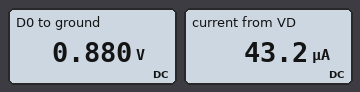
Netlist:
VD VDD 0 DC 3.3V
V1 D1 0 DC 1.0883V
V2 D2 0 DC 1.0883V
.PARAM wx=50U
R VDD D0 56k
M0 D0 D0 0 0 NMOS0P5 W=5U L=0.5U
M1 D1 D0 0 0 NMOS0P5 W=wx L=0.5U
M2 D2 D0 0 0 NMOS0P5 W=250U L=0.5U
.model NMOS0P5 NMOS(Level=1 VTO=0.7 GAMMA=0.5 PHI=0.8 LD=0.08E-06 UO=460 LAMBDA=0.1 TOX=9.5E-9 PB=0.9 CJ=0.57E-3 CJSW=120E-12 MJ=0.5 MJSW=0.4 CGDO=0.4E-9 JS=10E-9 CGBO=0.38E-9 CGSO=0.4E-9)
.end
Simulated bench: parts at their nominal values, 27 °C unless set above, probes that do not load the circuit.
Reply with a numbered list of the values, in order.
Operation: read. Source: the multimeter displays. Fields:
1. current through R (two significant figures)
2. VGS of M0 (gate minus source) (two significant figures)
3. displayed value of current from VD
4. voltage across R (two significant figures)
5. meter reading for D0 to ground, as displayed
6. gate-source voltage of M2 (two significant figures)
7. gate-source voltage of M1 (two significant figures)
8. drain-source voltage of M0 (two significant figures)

1. 43 µA
2. 880 mV
3. 43.2 µA
4. 2.4 V
5. 0.880 V
6. 880 mV
7. 880 mV
8. 880 mV
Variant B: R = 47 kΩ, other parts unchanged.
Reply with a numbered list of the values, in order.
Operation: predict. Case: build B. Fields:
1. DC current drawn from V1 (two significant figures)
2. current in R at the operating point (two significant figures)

1. 520 µA
2. 51 µA
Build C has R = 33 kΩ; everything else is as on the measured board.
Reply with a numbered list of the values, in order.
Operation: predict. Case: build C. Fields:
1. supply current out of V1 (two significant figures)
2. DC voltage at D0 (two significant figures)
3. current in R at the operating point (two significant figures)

1. 730 µA
2. 930 mV
3. 72 µA
